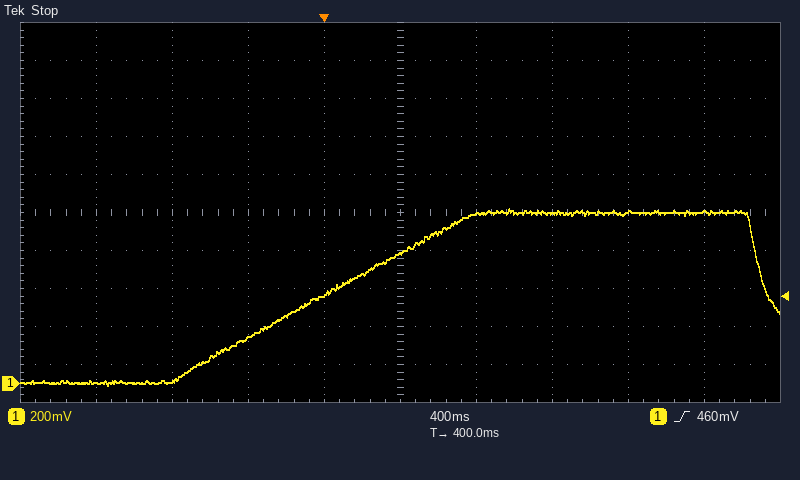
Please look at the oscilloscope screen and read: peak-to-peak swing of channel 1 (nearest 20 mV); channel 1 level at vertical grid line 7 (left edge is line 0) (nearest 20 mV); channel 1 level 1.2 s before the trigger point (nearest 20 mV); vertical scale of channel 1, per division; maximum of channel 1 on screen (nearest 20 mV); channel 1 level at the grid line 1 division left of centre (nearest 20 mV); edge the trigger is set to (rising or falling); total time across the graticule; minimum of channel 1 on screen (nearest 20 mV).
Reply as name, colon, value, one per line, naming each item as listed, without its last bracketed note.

peak-to-peak swing of channel 1: 940 mV
channel 1 level at vertical grid line 7 (left edge is line 0): 900 mV
channel 1 level 1.2 s before the trigger point: 0 mV
vertical scale of channel 1, per division: 200 mV
maximum of channel 1 on screen: 920 mV
channel 1 level at the grid line 1 division left of centre: 480 mV
edge the trigger is set to: rising
total time across the graticule: 4 s
minimum of channel 1 on screen: -20 mV
